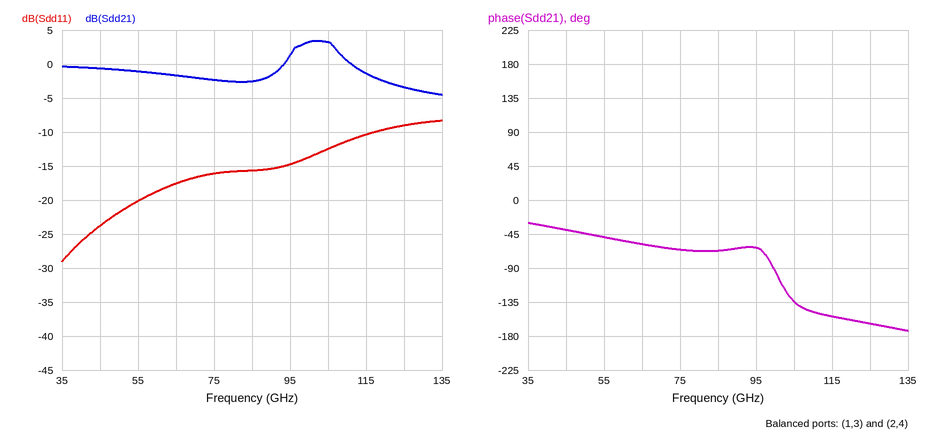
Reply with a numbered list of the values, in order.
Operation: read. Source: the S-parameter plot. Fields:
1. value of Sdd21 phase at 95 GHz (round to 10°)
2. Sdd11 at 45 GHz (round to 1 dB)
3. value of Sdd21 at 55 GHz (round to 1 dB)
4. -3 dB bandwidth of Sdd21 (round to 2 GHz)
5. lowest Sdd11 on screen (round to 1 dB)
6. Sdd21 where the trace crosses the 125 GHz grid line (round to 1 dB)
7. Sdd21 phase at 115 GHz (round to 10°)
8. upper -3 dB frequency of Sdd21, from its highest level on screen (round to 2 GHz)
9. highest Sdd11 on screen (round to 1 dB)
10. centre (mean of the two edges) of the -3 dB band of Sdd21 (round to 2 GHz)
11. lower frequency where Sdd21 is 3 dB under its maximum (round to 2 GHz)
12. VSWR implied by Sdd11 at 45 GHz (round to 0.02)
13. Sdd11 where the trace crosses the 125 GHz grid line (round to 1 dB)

1. -60°
2. -24 dB
3. -1 dB
4. 16 GHz
5. -29 dB
6. -3 dB
7. -150°
8. 110 GHz
9. -8 dB
10. 102 GHz
11. 94 GHz
12. 1.14
13. -9 dB
